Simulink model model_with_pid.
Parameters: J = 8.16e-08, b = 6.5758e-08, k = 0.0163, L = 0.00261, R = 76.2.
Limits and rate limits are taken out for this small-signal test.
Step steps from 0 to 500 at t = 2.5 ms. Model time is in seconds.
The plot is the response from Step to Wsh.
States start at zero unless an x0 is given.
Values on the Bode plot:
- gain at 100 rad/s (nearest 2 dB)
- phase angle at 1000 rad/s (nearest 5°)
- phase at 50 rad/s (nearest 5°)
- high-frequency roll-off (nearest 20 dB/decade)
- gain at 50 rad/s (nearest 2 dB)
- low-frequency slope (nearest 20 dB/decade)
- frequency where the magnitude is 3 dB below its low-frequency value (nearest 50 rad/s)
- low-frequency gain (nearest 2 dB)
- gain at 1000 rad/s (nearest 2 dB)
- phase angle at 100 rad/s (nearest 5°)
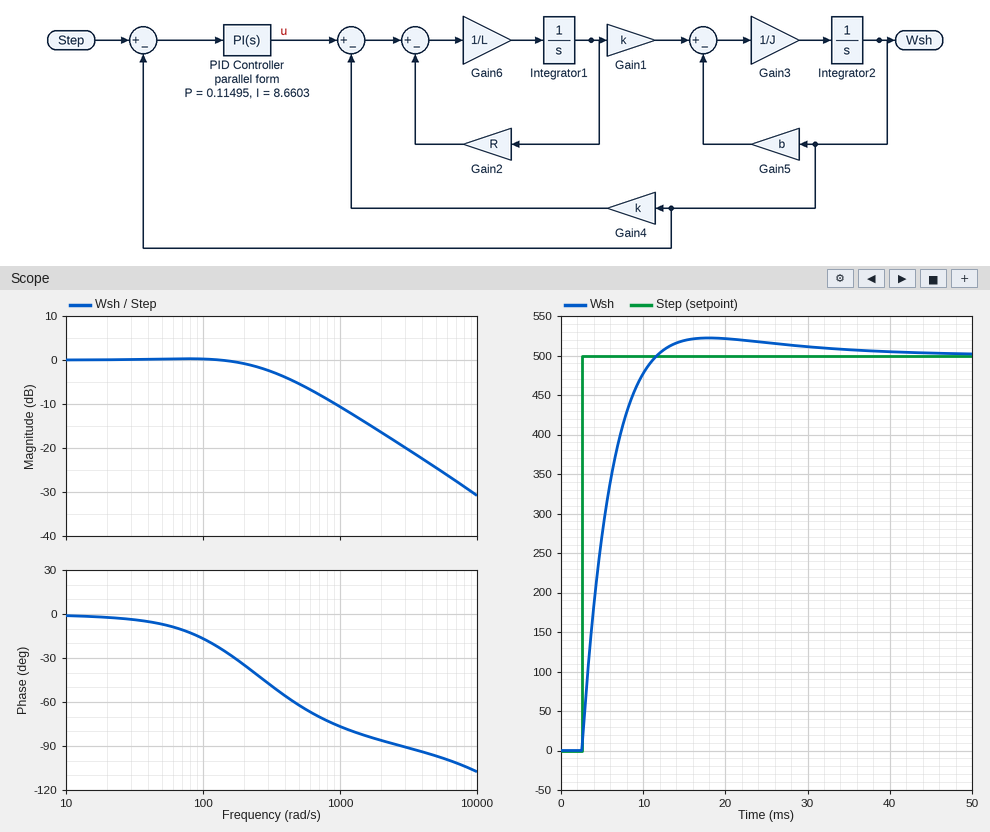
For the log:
0 dB
-75°
-5°
-20 dB/decade
0 dB
0 dB/decade
350 rad/s
0 dB
-10 dB
-15°
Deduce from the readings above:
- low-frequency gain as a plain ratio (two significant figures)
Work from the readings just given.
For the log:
1.0
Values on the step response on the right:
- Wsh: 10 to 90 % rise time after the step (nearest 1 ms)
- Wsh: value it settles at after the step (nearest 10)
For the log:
6 ms
500
